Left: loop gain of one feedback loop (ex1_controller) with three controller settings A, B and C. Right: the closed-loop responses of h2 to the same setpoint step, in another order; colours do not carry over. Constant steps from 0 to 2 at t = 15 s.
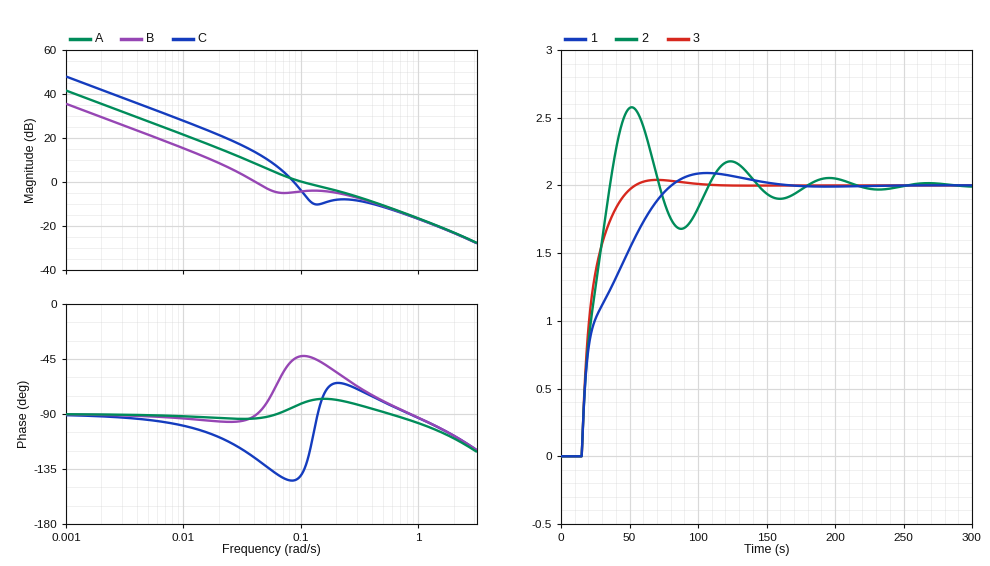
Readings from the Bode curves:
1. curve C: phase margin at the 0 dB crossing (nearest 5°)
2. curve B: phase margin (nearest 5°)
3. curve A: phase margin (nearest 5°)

35°
90°
100°
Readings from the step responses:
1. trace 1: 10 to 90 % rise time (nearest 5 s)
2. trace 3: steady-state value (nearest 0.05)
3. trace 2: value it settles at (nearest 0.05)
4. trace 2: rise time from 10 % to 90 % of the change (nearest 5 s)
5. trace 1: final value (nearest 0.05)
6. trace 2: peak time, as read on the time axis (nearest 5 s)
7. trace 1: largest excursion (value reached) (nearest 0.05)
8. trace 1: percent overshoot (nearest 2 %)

50 s
2.00
2.00
15 s
2.00
50 s
2.10
4 %
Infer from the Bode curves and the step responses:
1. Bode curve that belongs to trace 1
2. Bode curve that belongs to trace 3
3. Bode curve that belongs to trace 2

B
A
C
